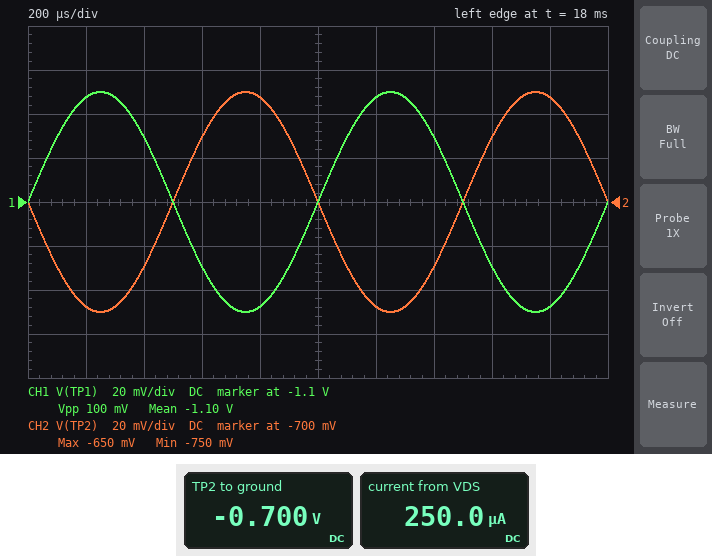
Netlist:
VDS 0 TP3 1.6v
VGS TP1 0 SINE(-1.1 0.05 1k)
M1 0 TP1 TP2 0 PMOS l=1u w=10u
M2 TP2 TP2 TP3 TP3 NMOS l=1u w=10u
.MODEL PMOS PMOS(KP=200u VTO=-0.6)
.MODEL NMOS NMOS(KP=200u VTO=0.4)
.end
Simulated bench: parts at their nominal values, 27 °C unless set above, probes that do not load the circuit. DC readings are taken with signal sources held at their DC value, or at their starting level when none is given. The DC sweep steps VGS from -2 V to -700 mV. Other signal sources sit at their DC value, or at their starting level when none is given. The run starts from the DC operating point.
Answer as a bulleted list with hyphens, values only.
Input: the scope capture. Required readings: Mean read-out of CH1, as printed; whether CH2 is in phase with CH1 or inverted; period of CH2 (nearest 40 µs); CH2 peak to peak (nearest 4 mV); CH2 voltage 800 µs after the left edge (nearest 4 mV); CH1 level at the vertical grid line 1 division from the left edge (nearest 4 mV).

- -1.10 V
- inverted
- 1.00 ms
- 100 mV
- -652 mV
- -1.052 V
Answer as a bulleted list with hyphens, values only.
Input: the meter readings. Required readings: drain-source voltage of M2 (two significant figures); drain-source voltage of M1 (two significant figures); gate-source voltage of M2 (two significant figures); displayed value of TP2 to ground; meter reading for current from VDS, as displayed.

- 900 mV
- 700 mV
- 900 mV
- -0.700 V
- 250.0 µA
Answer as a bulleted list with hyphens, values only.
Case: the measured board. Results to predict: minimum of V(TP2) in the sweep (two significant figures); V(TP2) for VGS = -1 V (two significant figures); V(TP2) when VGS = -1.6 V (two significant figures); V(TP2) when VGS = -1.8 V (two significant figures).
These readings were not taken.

- -1.1 V
- -800 mV
- -400 mV
- -350 mV
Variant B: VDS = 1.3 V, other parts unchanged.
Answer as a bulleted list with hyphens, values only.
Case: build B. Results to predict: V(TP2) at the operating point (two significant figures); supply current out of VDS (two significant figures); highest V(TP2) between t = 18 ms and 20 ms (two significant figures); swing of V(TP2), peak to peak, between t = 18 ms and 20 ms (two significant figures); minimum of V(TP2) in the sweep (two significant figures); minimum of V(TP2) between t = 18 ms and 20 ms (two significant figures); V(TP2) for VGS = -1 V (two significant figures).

- -410 mV
- 240 µA
- -380 mV
- 72 mV
- -800 mV
- -450 mV
- -500 mV
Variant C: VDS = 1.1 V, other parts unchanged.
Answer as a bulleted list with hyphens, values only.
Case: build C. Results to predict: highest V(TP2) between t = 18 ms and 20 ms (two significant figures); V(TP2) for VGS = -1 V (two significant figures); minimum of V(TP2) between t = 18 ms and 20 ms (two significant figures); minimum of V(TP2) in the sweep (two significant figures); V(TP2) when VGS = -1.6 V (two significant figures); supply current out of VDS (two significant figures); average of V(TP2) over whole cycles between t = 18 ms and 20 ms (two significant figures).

- -240 mV
- -310 mV
- -280 mV
- -600 mV
- -160 mV
- 190 µA
- -260 mV
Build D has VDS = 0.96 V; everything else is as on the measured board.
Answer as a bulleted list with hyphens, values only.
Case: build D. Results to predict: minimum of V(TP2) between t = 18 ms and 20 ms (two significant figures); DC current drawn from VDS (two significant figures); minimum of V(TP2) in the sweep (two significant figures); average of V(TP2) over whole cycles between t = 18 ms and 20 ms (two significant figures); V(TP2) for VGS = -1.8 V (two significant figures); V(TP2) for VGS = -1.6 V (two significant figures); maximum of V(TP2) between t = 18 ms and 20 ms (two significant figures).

- -190 mV
- 150 µA
- -460 mV
- -180 mV
- -94 mV
- -110 mV
- -170 mV
